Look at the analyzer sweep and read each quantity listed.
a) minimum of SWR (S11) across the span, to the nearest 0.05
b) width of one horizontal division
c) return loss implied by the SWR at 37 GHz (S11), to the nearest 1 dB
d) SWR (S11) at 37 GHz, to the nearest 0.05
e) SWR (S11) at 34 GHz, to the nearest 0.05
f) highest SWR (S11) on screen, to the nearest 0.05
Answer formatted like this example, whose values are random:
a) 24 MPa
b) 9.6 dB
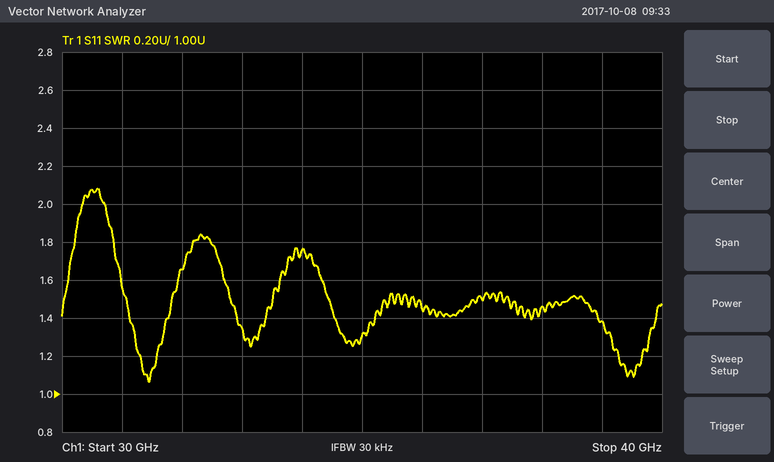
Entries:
a) 1.05
b) 1 GHz
c) 14 dB
d) 1.50
e) 1.75
f) 2.10
